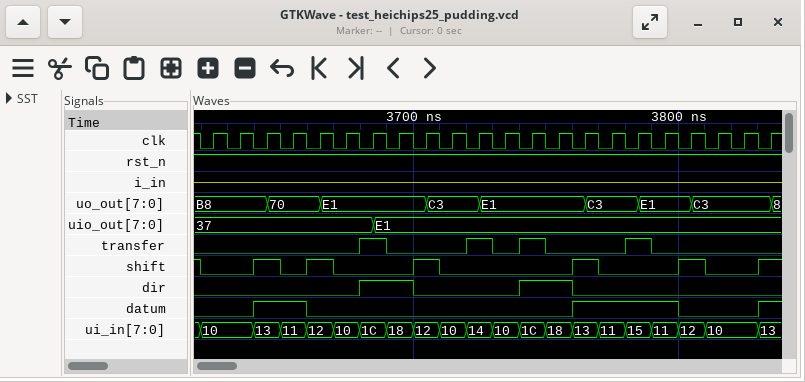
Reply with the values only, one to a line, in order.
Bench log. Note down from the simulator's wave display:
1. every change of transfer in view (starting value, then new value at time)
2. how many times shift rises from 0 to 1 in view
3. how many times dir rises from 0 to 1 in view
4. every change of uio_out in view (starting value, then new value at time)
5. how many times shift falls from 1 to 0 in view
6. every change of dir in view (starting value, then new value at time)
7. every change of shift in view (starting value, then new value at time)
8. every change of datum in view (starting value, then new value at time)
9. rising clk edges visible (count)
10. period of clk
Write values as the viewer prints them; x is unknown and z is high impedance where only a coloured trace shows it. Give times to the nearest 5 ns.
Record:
0, 1 at 3680 ns, 0 at 3690 ns, 1 at 3720 ns, 0 at 3730 ns, 1 at 3740 ns, 0 at 3750 ns, 1 at 3780 ns, 0 at 3790 ns
6
2
37, E1 at 3685 ns
6
0, 1 at 3680 ns, 0 at 3700 ns, 1 at 3740 ns, 0 at 3760 ns
1, 0 at 3620 ns, 1 at 3640 ns, 0 at 3650 ns, 1 at 3660 ns, 0 at 3670 ns, 1 at 3700 ns, 0 at 3710 ns, 1 at 3760 ns, 0 at 3770 ns, 1 at 3800 ns, 0 at 3810 ns, 1 at 3830 ns
0, 1 at 3640 ns, 0 at 3660 ns, 1 at 3760 ns, 0 at 3800 ns, 1 at 3830 ns
22
10 ns
